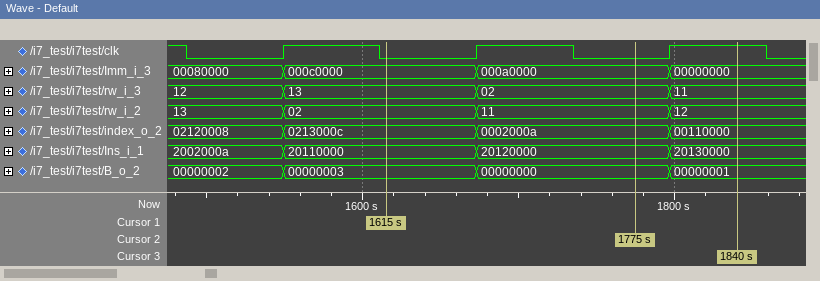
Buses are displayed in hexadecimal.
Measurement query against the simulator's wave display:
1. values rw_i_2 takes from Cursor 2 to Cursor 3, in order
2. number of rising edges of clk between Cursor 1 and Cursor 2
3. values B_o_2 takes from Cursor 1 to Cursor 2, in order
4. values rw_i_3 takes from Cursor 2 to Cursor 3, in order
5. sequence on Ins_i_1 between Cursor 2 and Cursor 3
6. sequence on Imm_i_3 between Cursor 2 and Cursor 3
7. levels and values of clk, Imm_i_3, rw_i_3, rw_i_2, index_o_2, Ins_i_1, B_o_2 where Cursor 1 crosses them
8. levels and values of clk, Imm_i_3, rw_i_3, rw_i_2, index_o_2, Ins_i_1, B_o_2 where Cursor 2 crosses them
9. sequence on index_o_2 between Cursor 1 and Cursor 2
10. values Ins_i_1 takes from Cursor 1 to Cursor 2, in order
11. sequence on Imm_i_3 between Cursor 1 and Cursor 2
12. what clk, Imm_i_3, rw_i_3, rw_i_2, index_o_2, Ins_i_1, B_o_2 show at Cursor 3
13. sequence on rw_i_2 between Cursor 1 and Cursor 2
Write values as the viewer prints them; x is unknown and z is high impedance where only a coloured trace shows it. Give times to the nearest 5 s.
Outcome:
11, 12
1
00000003, 00000000
02, 11
20120000, 20130000
000a0000, 00000000
clk=0, Imm_i_3=000c0000, rw_i_3=13, rw_i_2=02, index_o_2=0213000c, Ins_i_1=20110000, B_o_2=00000003
clk=0, Imm_i_3=000a0000, rw_i_3=02, rw_i_2=11, index_o_2=0002000a, Ins_i_1=20120000, B_o_2=00000000
0213000c, 0002000a
20110000, 20120000
000c0000, 000a0000
clk=1, Imm_i_3=00000000, rw_i_3=11, rw_i_2=12, index_o_2=00110000, Ins_i_1=20130000, B_o_2=00000001
02, 11
